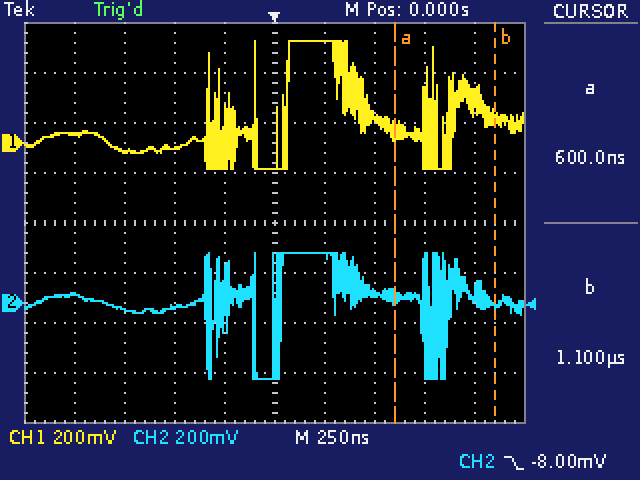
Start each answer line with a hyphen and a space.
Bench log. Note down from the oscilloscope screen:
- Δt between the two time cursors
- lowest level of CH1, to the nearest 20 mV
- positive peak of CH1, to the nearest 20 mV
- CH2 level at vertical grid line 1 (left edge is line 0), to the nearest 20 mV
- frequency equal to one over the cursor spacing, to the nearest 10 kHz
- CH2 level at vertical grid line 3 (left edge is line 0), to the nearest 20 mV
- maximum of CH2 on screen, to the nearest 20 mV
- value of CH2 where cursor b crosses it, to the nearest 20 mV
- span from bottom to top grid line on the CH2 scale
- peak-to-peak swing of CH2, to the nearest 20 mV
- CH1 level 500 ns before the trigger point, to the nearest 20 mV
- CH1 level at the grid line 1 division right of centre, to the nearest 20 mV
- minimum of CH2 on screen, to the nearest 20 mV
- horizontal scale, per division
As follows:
- 500 ns
- -100 mV
- 400 mV
- 40 mV
- 2.00 MHz
- -20 mV
- 200 mV
- 0 mV
- 1.6 V
- 500 mV
- -20 mV
- 400 mV
- -300 mV
- 250 ns
